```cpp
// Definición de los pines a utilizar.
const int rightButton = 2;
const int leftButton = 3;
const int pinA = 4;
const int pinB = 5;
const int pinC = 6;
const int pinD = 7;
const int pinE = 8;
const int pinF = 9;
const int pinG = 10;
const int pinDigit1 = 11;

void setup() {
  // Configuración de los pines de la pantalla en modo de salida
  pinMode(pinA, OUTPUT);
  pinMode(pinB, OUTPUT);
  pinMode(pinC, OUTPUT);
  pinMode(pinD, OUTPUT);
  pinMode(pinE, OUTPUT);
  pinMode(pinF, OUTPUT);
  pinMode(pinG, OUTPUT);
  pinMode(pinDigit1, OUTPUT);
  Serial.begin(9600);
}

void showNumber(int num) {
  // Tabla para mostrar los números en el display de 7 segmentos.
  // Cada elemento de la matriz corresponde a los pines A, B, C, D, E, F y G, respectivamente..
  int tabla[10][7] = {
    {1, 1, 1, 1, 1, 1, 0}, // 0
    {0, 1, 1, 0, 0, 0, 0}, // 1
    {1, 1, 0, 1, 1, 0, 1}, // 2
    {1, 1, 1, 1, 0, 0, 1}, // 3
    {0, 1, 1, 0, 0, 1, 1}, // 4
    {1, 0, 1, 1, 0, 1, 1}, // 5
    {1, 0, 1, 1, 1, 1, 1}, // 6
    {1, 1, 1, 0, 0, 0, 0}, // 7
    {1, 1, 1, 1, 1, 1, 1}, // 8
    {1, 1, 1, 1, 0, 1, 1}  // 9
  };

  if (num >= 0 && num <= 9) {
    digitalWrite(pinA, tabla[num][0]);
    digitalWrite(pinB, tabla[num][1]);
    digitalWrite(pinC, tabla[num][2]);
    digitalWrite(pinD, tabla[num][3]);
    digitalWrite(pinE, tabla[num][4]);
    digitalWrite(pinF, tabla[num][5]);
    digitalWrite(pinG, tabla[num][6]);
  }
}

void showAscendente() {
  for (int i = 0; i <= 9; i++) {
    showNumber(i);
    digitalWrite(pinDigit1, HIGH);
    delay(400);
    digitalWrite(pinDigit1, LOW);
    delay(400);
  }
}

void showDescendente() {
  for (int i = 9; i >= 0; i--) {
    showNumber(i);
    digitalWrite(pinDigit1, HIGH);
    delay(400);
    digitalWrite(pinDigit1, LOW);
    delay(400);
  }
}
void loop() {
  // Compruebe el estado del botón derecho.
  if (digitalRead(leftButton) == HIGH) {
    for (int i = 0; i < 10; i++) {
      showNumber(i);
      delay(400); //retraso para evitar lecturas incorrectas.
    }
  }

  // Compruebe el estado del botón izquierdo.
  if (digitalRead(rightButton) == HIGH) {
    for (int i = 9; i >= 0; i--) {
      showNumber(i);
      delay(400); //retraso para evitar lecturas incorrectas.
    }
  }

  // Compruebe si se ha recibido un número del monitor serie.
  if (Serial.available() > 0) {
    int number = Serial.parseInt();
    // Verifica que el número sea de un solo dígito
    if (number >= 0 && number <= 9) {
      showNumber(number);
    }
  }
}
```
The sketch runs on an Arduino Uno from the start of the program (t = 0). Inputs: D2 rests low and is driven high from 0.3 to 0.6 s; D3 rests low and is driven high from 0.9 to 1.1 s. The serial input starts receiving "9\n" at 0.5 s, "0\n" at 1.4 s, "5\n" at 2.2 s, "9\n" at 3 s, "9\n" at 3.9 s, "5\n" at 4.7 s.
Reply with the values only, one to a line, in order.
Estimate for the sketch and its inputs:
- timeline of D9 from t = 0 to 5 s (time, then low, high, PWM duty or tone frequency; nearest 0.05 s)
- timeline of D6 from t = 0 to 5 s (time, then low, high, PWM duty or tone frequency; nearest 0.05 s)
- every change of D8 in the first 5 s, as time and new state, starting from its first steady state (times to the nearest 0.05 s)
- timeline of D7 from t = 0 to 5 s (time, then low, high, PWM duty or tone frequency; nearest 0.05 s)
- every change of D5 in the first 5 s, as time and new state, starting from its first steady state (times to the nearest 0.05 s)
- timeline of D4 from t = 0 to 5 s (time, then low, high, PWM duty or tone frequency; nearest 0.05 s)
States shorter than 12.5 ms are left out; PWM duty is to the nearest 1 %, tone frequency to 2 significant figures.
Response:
0 s low; 0.3 s high; 1.1 s low; 1.5 s high; 2.7 s low; 3.9 s high
0 s low; 0.3 s high; 3.1 s low; 3.5 s high
0 s low; 0.7 s high; 1.1 s low; 1.5 s high; 1.9 s low; 3.1 s high; 3.5 s low; 3.9 s high; 4.3 s low
0 s low; 0.3 s high; 1.1 s low; 1.5 s high; 2.3 s low; 2.7 s high; 3.5 s low; 3.9 s high
0 s low; 0.3 s high; 1.5 s low; 2.3 s high; 4.7 s low
0 s low; 0.3 s high; 2.3 s low; 2.7 s high; 3.5 s low; 3.9 s high
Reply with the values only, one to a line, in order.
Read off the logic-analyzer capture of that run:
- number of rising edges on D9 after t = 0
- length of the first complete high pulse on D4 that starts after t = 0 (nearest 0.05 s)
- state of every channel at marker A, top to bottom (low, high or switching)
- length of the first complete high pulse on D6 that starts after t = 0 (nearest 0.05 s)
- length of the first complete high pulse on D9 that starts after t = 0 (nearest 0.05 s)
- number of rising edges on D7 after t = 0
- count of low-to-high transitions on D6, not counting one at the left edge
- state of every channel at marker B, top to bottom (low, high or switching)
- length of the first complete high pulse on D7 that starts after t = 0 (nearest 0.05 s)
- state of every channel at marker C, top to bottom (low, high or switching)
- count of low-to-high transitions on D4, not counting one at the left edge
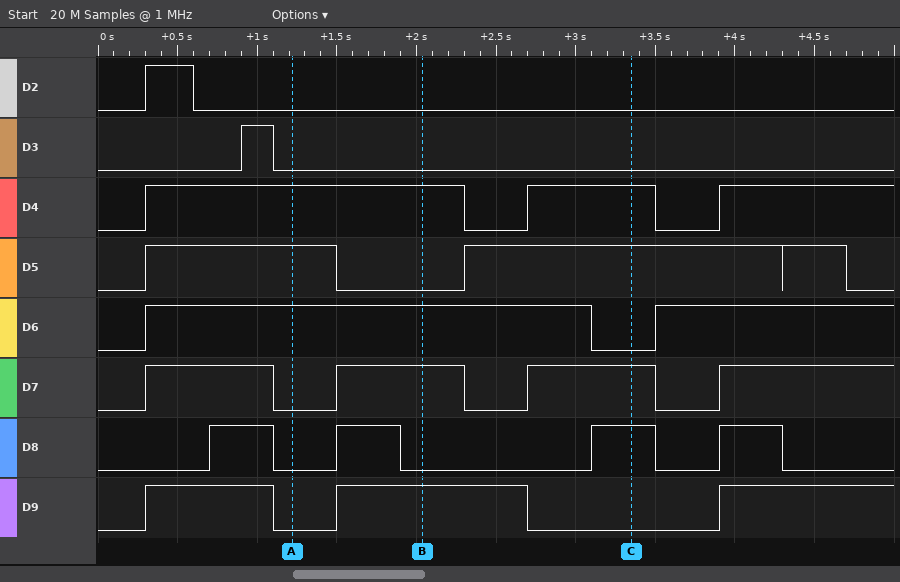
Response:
3
2.00 s
D2 low, D3 low, D4 high, D5 high, D6 high, D7 low, D8 low, D9 low
2.80 s
0.80 s
4
2
D2 low, D3 low, D4 high, D5 low, D6 high, D7 high, D8 low, D9 high
0.80 s
D2 low, D3 low, D4 high, D5 high, D6 low, D7 high, D8 high, D9 low
3
